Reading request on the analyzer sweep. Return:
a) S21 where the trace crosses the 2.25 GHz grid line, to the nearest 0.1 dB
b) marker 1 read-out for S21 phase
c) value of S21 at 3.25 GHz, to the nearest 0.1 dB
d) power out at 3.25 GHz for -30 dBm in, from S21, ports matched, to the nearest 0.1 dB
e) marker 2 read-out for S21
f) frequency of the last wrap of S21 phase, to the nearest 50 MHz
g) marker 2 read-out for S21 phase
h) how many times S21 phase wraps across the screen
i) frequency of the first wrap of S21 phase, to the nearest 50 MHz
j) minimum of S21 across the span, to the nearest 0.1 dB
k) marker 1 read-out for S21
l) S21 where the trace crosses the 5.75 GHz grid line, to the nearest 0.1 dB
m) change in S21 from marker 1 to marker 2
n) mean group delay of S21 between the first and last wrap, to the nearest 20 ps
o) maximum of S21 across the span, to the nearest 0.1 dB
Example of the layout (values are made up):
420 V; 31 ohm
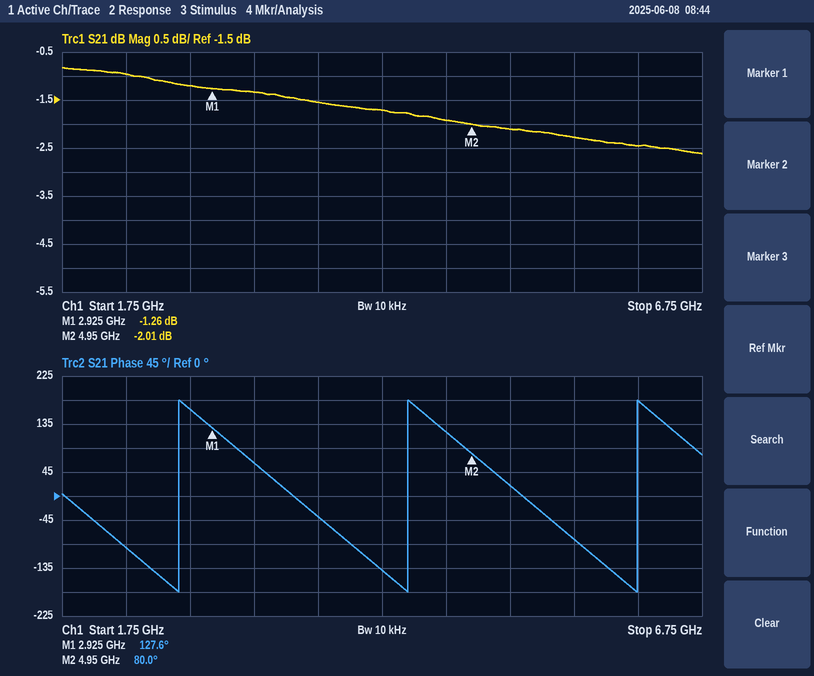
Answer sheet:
-1.0 dB; 127.6°; -1.3 dB; -31.3 dBm; -2.01 dB; 6.25 GHz; 80.0°; 3; 2.65 GHz; -2.6 dB; -1.26 dB; -2.3 dB; -0.75 dB; 560 ps; -0.8 dB
